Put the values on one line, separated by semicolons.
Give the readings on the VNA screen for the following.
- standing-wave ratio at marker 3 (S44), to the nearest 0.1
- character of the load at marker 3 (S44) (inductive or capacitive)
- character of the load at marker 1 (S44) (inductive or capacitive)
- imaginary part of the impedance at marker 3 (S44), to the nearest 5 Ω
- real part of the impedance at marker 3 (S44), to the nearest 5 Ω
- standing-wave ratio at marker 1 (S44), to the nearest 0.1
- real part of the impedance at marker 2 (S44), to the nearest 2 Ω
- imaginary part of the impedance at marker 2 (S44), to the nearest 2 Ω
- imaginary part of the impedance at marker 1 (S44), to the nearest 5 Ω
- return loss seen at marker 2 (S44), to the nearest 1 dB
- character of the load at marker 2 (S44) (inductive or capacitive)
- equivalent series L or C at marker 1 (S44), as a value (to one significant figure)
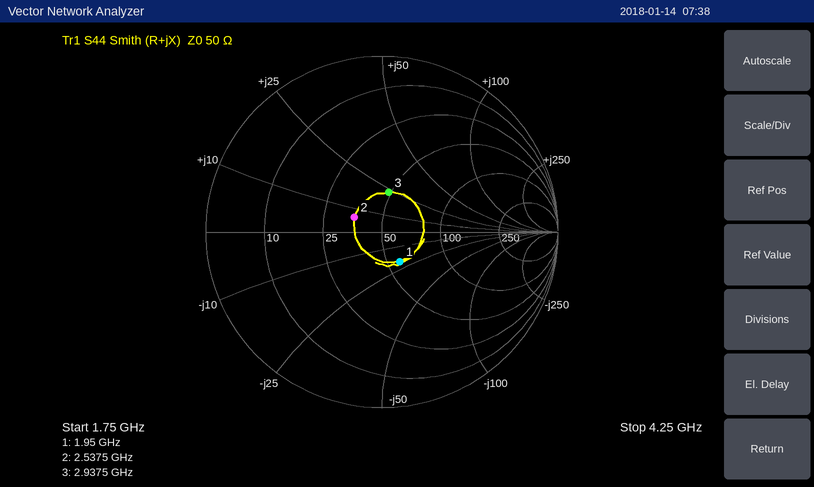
1.6; inductive; capacitive; +25 Ω; 50 Ω; 1.5; 36 Ω; +6 Ω; -20 Ω; 15 dB; inductive; 4 pF
